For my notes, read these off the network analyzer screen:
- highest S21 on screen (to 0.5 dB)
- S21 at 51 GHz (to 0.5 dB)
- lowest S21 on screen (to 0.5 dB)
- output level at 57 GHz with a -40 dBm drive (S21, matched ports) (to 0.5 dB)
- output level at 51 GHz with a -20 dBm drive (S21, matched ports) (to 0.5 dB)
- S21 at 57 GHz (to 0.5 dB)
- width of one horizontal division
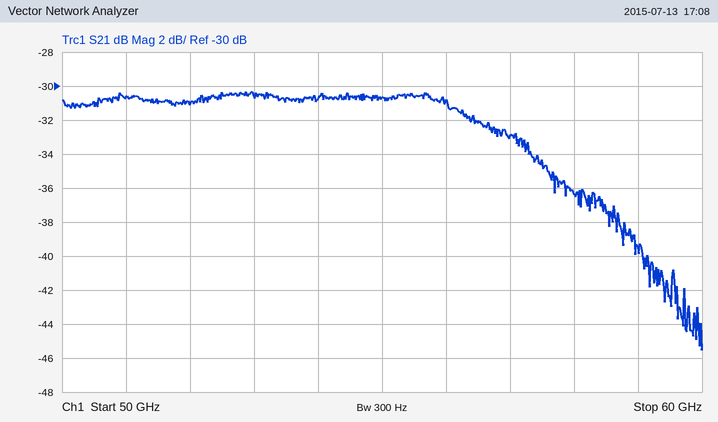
-30.5 dB
-30.5 dB
-45.5 dB
-73.0 dBm
-50.5 dBm
-33.0 dB
1 GHz
